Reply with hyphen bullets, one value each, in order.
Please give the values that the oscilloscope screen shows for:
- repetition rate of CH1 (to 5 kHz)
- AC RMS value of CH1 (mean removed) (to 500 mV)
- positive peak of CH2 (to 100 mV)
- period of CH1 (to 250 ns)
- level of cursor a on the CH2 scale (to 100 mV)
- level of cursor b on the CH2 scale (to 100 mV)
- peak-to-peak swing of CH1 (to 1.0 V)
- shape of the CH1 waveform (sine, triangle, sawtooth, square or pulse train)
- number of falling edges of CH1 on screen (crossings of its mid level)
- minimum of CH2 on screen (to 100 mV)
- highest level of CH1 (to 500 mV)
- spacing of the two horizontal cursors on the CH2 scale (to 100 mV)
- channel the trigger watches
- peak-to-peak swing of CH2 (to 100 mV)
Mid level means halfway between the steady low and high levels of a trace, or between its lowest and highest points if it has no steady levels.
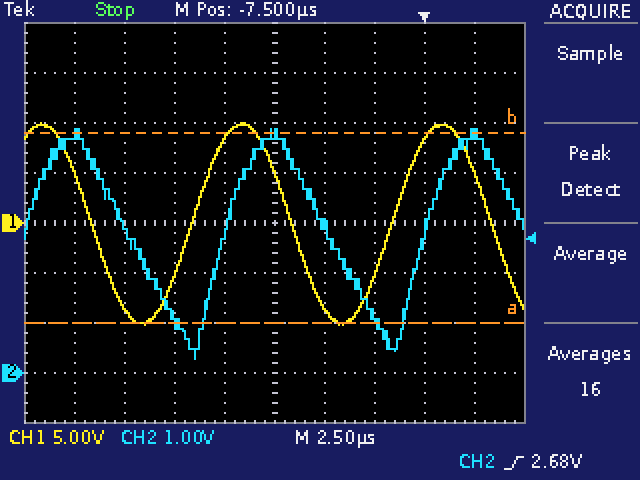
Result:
- 100 kHz
- 7.0 V
- 4.9 V
- 10.00 µs
- 1.0 V
- 4.8 V
- 20.0 V
- sine
- 3
- 300 mV
- 10.0 V
- 3.8 V
- CH2
- 4.6 V
